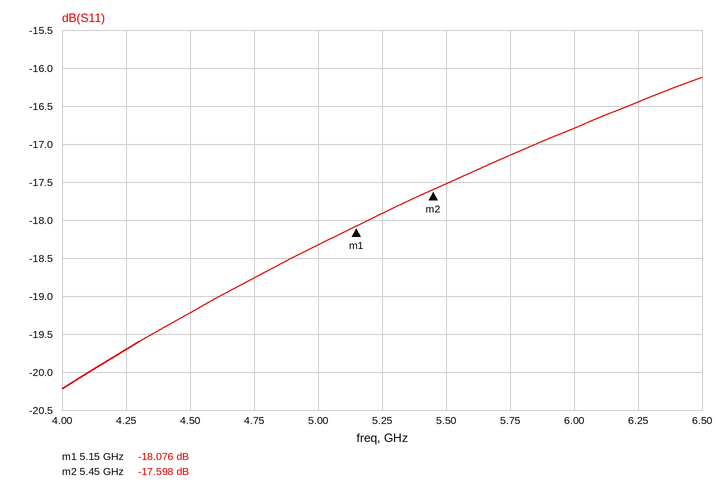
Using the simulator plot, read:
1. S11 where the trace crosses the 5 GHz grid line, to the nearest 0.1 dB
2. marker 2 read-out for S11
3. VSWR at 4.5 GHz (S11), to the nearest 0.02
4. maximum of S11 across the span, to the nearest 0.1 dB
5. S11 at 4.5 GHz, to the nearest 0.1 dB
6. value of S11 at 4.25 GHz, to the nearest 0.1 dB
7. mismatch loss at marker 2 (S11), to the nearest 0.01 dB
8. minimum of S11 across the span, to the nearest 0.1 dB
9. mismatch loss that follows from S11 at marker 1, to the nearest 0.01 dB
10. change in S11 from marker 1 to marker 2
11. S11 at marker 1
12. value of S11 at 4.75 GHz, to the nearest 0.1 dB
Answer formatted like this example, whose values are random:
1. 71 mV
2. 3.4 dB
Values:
1. -18.3 dB
2. -17.598 dB
3. 1.24
4. -16.1 dB
5. -19.2 dB
6. -19.7 dB
7. 0.08 dB
8. -20.2 dB
9. 0.07 dB
10. 0.478 dB
11. -18.076 dB
12. -18.8 dB
